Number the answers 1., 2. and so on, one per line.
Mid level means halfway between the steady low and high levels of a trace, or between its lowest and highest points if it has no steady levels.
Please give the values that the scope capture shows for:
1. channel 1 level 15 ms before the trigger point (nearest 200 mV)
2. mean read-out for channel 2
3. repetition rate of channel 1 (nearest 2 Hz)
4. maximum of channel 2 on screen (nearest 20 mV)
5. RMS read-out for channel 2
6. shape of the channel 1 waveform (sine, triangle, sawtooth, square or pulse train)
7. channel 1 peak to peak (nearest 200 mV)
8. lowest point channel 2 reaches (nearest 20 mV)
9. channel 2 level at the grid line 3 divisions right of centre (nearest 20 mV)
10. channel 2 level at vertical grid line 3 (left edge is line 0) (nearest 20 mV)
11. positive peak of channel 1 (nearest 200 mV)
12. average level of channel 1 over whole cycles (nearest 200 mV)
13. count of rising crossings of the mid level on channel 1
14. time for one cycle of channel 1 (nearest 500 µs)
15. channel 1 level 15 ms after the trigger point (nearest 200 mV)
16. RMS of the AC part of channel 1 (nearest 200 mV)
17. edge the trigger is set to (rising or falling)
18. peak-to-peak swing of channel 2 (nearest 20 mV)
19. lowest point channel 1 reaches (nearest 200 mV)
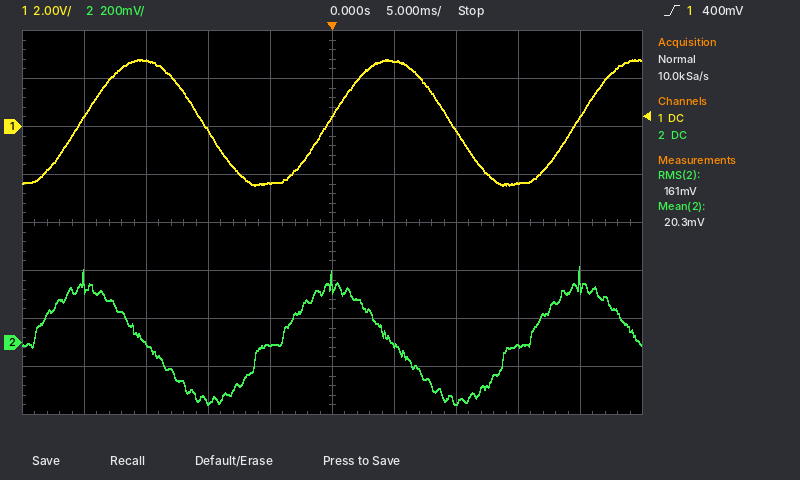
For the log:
1. 2.8 V
2. 20.3 mV
3. 50 Hz
4. 320 mV
5. 161 mV
6. sine
7. 5.2 V
8. -260 mV
9. -20 mV
10. -240 mV
11. 2.8 V
12. 200 mV
13. 3
14. 20.0 ms
15. -2.4 V
16. 1.8 V
17. rising
18. 580 mV
19. -2.4 V
